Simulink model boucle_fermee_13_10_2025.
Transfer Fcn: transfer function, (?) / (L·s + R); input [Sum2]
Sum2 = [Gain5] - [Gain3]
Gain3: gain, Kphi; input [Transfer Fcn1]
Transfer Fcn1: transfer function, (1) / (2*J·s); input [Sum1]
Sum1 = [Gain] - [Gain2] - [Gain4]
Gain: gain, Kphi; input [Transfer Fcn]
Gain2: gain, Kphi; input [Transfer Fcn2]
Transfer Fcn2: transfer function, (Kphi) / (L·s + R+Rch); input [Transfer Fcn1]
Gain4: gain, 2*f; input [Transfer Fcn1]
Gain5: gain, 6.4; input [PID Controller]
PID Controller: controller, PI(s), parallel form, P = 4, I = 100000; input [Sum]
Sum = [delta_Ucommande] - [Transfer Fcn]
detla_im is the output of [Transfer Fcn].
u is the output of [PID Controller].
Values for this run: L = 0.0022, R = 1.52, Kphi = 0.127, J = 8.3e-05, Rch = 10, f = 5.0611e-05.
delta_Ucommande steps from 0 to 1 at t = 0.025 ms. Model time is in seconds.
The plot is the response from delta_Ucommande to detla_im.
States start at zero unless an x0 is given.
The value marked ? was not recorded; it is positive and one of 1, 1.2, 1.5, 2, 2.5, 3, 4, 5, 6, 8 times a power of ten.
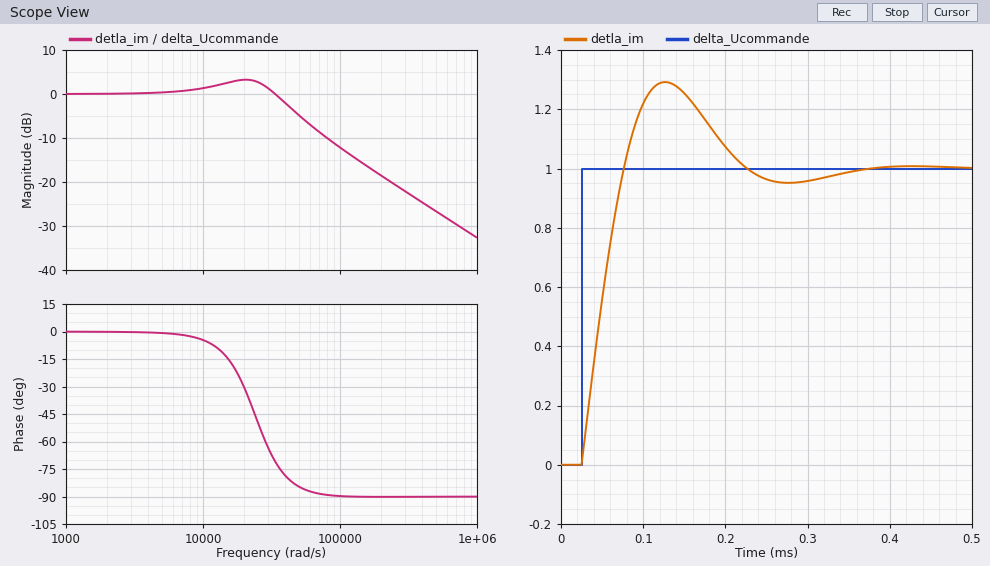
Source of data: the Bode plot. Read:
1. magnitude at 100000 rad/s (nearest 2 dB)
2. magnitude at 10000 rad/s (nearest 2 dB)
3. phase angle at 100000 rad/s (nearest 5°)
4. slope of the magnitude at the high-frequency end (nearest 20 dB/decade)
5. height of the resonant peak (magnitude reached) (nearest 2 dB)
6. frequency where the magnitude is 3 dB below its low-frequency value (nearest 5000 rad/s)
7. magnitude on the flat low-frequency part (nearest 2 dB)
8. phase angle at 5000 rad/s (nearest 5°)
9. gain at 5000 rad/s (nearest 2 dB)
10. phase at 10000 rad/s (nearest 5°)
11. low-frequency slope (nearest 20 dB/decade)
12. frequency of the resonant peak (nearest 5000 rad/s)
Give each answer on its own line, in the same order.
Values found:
-12 dB
2 dB
-90°
-20 dB/decade
4 dB
45000 rad/s
0 dB
0°
0 dB
-5°
0 dB/decade
20000 rad/s
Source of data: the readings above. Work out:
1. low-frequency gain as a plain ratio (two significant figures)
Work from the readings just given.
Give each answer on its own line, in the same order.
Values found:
1.0
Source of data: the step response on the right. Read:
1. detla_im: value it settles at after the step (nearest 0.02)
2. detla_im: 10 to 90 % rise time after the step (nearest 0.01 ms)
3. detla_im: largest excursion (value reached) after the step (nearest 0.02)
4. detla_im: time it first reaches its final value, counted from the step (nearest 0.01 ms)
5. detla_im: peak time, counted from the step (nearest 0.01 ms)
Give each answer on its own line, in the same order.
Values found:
1.00
0.04 ms
1.30
0.05 ms
0.10 ms
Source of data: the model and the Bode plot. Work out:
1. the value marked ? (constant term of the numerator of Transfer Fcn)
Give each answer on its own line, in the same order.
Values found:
2
